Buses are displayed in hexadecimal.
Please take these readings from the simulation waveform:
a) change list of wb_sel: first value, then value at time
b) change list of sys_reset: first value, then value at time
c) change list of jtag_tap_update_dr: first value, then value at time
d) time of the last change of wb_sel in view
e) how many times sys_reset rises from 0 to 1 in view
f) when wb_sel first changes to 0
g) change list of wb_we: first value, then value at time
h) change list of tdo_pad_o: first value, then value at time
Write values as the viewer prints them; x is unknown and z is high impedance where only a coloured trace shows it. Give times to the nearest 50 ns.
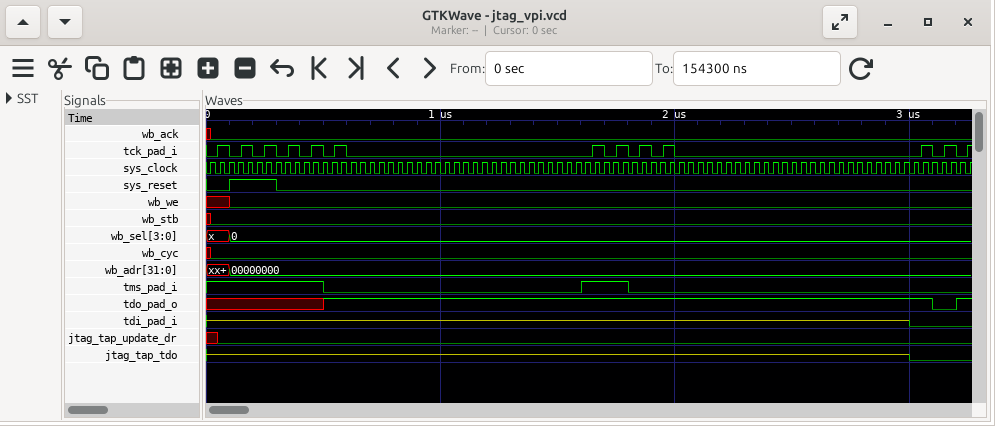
x, 0 at 100 ns
0, 1 at 100 ns, 0 at 300 ns
x, 0 at 50 ns
100 ns
1
100 ns
x, 0 at 100 ns
x, 1 at 500 ns, 0 at 3100 ns, 1 at 3200 ns
